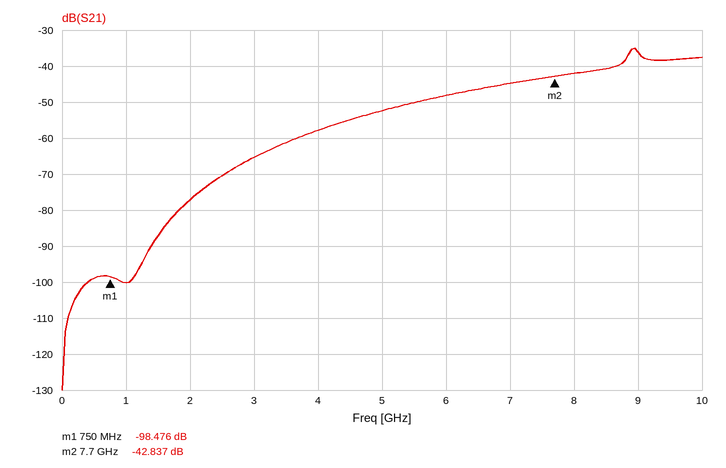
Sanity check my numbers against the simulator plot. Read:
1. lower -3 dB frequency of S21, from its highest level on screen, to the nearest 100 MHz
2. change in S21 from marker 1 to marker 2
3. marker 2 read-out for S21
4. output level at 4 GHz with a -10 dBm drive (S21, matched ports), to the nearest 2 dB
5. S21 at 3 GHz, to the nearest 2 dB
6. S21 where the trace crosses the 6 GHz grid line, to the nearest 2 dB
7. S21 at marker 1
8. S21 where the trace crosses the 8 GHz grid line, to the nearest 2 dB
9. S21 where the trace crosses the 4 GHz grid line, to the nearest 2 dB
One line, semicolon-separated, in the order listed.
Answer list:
8.8 GHz; 55.639 dB; -42.837 dB; -68 dBm; -66 dB; -48 dB; -98.476 dB; -42 dB; -58 dB
